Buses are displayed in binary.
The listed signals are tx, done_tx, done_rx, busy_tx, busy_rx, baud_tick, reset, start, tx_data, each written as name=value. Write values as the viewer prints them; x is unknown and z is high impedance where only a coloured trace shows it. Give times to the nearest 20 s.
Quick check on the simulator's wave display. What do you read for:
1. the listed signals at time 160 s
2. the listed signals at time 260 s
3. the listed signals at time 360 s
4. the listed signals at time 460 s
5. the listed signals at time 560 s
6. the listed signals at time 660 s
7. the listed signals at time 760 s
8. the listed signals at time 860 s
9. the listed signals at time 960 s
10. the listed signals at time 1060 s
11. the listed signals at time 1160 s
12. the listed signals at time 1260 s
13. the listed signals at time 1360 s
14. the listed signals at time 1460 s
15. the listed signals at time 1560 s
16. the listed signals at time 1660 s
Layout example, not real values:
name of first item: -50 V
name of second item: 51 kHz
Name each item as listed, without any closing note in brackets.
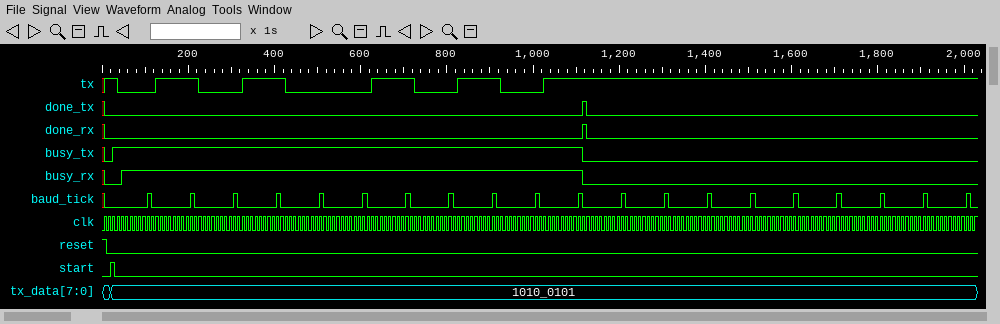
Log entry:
the listed signals at time 160 s: tx=1, done_tx=0, done_rx=0, busy_tx=1, busy_rx=1, baud_tick=0, reset=0, start=0, tx_data=1010_0101
the listed signals at time 260 s: tx=0, done_tx=0, done_rx=0, busy_tx=1, busy_rx=1, baud_tick=0, reset=0, start=0, tx_data=1010_0101
the listed signals at time 360 s: tx=1, done_tx=0, done_rx=0, busy_tx=1, busy_rx=1, baud_tick=0, reset=0, start=0, tx_data=1010_0101
the listed signals at time 460 s: tx=0, done_tx=0, done_rx=0, busy_tx=1, busy_rx=1, baud_tick=0, reset=0, start=0, tx_data=1010_0101
the listed signals at time 560 s: tx=0, done_tx=0, done_rx=0, busy_tx=1, busy_rx=1, baud_tick=0, reset=0, start=0, tx_data=1010_0101
the listed signals at time 660 s: tx=1, done_tx=0, done_rx=0, busy_tx=1, busy_rx=1, baud_tick=0, reset=0, start=0, tx_data=1010_0101
the listed signals at time 760 s: tx=0, done_tx=0, done_rx=0, busy_tx=1, busy_rx=1, baud_tick=0, reset=0, start=0, tx_data=1010_0101
the listed signals at time 860 s: tx=1, done_tx=0, done_rx=0, busy_tx=1, busy_rx=1, baud_tick=0, reset=0, start=0, tx_data=1010_0101
the listed signals at time 960 s: tx=0, done_tx=0, done_rx=0, busy_tx=1, busy_rx=1, baud_tick=0, reset=0, start=0, tx_data=1010_0101
the listed signals at time 1060 s: tx=1, done_tx=0, done_rx=0, busy_tx=1, busy_rx=1, baud_tick=0, reset=0, start=0, tx_data=1010_0101
the listed signals at time 1160 s: tx=1, done_tx=0, done_rx=0, busy_tx=0, busy_rx=0, baud_tick=0, reset=0, start=0, tx_data=1010_0101
the listed signals at time 1260 s: tx=1, done_tx=0, done_rx=0, busy_tx=0, busy_rx=0, baud_tick=0, reset=0, start=0, tx_data=1010_0101
the listed signals at time 1360 s: tx=1, done_tx=0, done_rx=0, busy_tx=0, busy_rx=0, baud_tick=0, reset=0, start=0, tx_data=1010_0101
the listed signals at time 1460 s: tx=1, done_tx=0, done_rx=0, busy_tx=0, busy_rx=0, baud_tick=0, reset=0, start=0, tx_data=1010_0101
the listed signals at time 1560 s: tx=1, done_tx=0, done_rx=0, busy_tx=0, busy_rx=0, baud_tick=0, reset=0, start=0, tx_data=1010_0101
the listed signals at time 1660 s: tx=1, done_tx=0, done_rx=0, busy_tx=0, busy_rx=0, baud_tick=0, reset=0, start=0, tx_data=1010_0101
